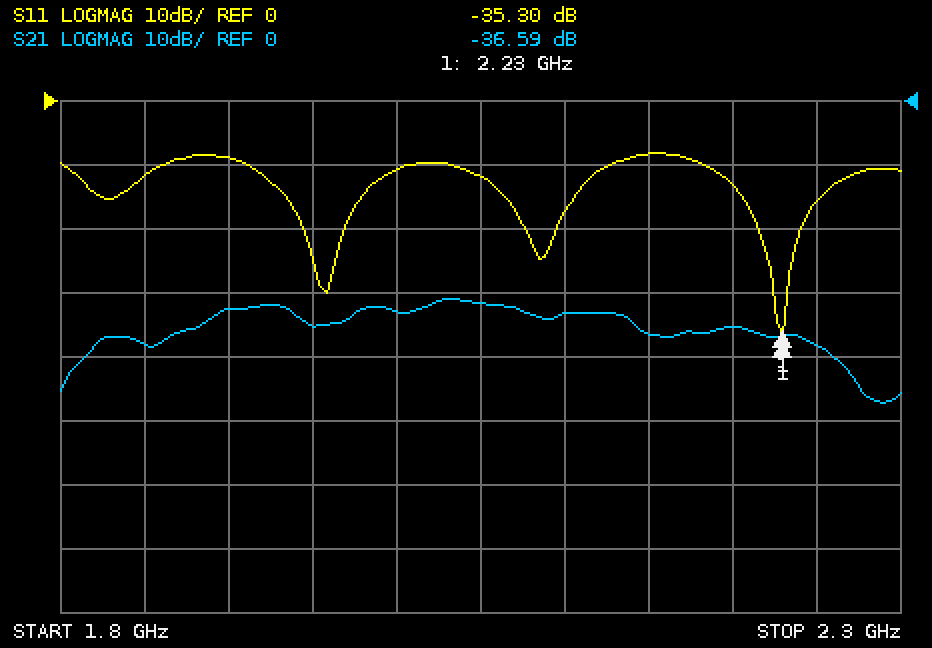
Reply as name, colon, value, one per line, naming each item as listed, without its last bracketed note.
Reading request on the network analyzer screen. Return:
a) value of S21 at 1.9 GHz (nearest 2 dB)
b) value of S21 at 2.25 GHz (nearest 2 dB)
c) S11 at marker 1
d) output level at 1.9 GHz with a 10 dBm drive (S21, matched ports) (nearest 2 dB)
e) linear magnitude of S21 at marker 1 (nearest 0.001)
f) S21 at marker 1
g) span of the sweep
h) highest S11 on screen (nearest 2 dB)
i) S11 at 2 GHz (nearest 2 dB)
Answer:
value of S21 at 1.9 GHz: -32 dB
value of S21 at 2.25 GHz: -38 dB
S11 at marker 1: -35.30 dB
output level at 1.9 GHz with a 10 dBm drive (S21, matched ports): -22 dBm
linear magnitude of S21 at marker 1: 0.015
S21 at marker 1: -36.59 dB
span of the sweep: 500 MHz
highest S11 on screen: -8 dB
S11 at 2 GHz: -10 dB
